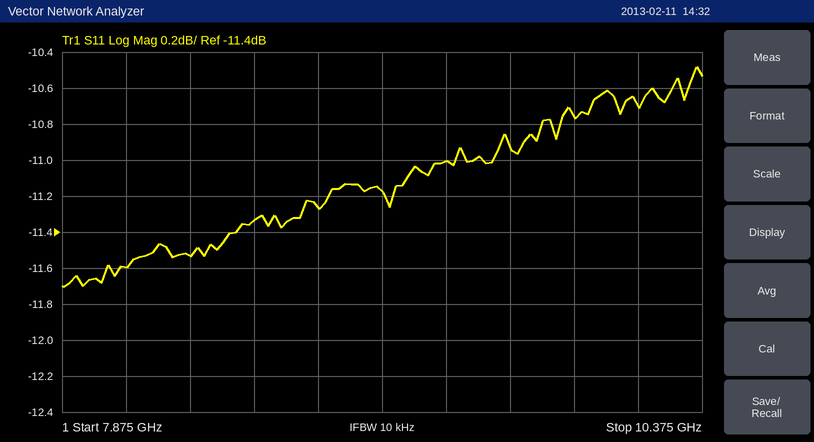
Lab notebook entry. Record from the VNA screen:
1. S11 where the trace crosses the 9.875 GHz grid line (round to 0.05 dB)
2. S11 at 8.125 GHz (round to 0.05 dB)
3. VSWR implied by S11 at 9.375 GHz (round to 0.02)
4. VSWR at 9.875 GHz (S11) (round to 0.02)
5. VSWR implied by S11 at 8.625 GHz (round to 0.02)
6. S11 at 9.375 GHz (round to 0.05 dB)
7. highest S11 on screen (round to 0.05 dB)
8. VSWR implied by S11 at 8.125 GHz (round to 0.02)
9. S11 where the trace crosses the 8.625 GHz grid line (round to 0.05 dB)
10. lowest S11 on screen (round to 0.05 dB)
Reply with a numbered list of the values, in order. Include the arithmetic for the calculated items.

1. -10.75 dB
2. -11.60 dB
3. |Γ| = 10^(-11/20) = 0.2818; VSWR = (1 + 0.2818)/(1 − 0.2818) ≈ 1.78
4. |Γ| = 10^(-10.75/20) = 0.2901; VSWR = (1 + 0.2901)/(1 − 0.2901) ≈ 1.82
5. |Γ| = 10^(-11.35/20) = 0.2707; VSWR = (1 + 0.2707)/(1 − 0.2707) ≈ 1.74
6. -11.00 dB
7. -10.50 dB
8. |Γ| = 10^(-11.6/20) = 0.2630; VSWR = (1 + 0.2630)/(1 − 0.2630) ≈ 1.71, so 1.72 to the nearest 0.02
9. -11.35 dB
10. -11.70 dB
